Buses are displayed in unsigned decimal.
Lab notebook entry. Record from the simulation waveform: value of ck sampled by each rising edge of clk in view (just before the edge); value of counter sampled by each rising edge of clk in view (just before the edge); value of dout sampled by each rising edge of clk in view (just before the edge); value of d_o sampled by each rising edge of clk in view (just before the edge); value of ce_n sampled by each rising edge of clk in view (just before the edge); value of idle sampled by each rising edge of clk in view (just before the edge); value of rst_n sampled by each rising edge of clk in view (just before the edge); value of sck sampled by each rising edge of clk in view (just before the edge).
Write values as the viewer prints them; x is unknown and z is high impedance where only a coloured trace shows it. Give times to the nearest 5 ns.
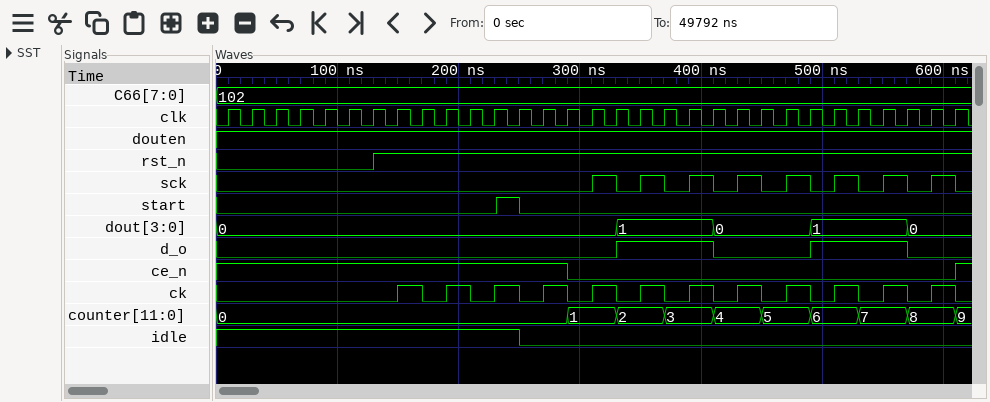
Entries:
0 0 0 0 0 0 0 0 1 0 1 0 1 0 1 0 1 0 1 0 1 0 1 0 1 0 1 0 1 0 1
0, 0, 0, 0, 0, 0, 0, 0, 0, 0, 0, 0, 0, 0, 0, 1, 1, 2, 2, 3, 3, 4, 4, 5, 5, 6, 6, 7, 7, 8, 8
0, 0, 0, 0, 0, 0, 0, 0, 0, 0, 0, 0, 0, 0, 0, 0, 0, 1, 1, 1, 1, 0, 0, 0, 0, 1, 1, 1, 1, 0, 0
0 0 0 0 0 0 0 0 0 0 0 0 0 0 0 0 0 1 1 1 1 0 0 0 0 1 1 1 1 0 0
1 1 1 1 1 1 1 1 1 1 1 1 1 1 1 0 0 0 0 0 0 0 0 0 0 0 0 0 0 0 0
1 1 1 1 1 1 1 1 1 1 1 1 1 0 0 0 0 0 0 0 0 0 0 0 0 0 0 0 0 0 0
0 0 0 0 0 0 0 1 1 1 1 1 1 1 1 1 1 1 1 1 1 1 1 1 1 1 1 1 1 1 1
0 0 0 0 0 0 0 0 0 0 0 0 0 0 0 0 1 0 1 0 1 0 1 0 1 0 1 0 1 0 1
